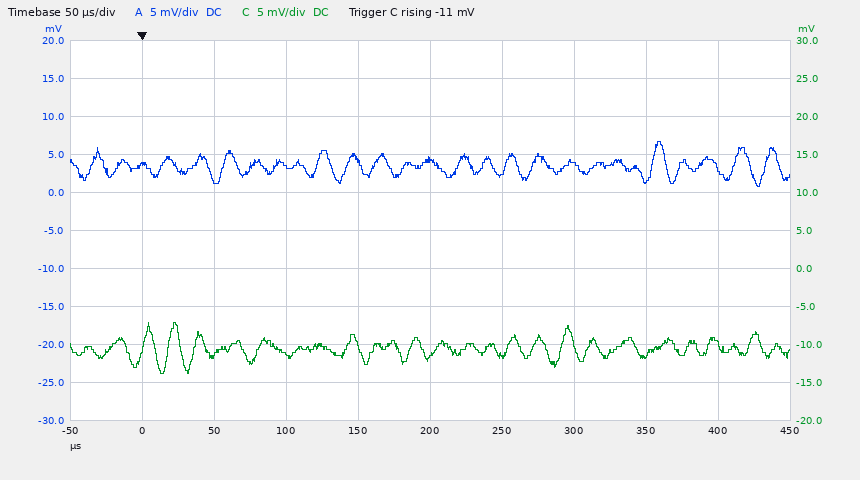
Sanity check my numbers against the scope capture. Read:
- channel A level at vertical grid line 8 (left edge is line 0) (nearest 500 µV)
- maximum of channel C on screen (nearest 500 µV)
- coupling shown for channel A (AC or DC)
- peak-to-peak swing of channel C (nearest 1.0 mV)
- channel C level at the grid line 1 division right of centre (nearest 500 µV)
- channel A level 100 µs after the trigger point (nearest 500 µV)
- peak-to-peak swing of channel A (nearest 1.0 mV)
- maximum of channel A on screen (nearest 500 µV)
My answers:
1.5 mV
-7.0 mV
DC
7.0 mV
-11.5 mV
3.5 mV
6.0 mV
6.5 mV
